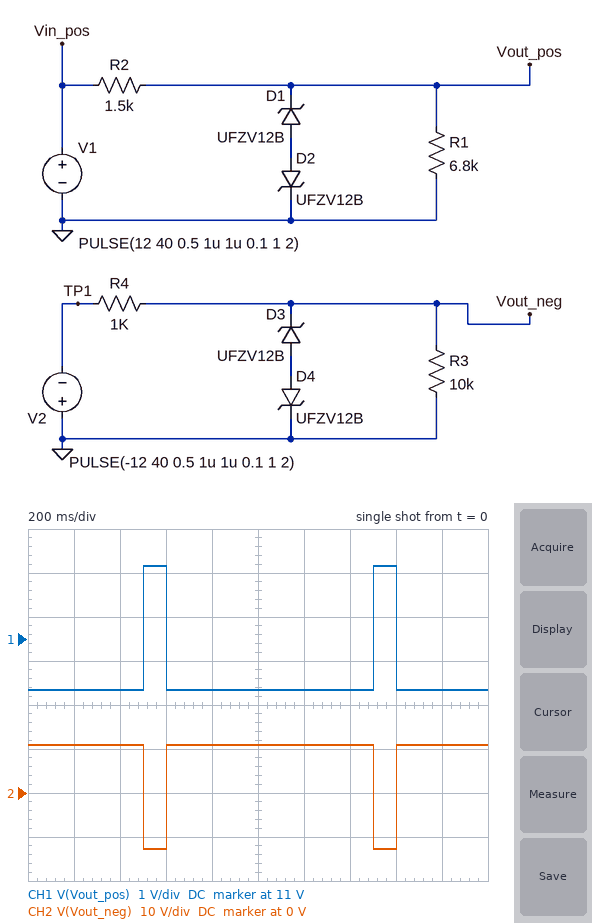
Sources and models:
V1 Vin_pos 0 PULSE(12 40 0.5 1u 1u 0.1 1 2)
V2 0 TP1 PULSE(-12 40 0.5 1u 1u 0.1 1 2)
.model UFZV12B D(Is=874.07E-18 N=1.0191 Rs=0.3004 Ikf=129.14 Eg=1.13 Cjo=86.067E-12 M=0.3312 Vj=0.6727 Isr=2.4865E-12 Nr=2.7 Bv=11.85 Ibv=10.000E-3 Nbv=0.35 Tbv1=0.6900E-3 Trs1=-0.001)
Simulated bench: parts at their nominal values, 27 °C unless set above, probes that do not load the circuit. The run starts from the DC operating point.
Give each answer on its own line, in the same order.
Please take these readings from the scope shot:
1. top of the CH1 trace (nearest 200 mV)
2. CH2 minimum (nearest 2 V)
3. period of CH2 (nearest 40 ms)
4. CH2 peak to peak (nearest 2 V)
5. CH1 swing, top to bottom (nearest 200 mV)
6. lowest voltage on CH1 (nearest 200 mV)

12.6 V
-12 V
1.00 s
24 V
2.8 V
9.8 V
